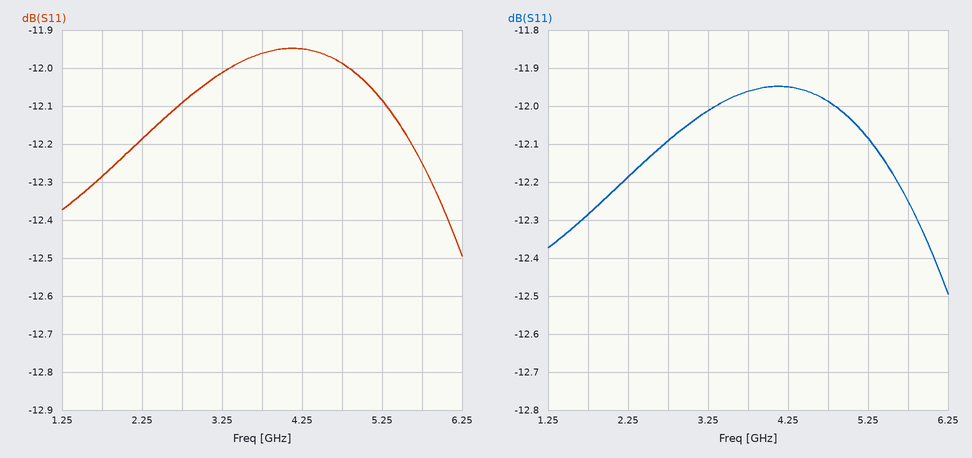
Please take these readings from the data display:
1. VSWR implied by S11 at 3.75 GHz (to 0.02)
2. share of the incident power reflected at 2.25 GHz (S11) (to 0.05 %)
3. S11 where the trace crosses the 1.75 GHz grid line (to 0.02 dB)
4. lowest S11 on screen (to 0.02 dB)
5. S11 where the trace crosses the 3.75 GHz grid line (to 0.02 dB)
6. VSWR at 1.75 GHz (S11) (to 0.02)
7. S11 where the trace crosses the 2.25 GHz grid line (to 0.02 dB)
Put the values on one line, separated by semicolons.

1.68; 6.05 %; -12.28 dB; -12.50 dB; -11.96 dB; 1.64; -12.18 dB
